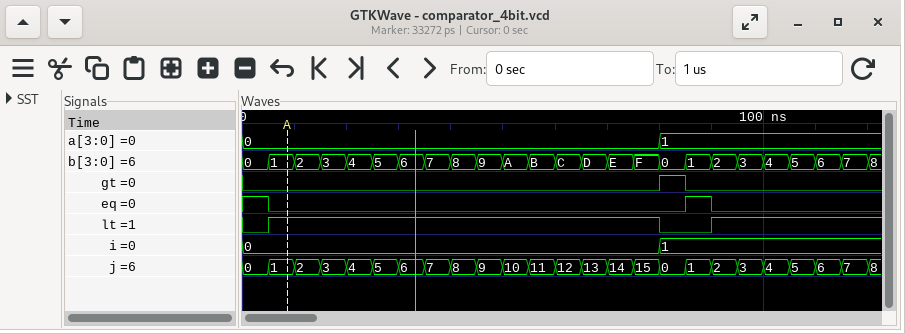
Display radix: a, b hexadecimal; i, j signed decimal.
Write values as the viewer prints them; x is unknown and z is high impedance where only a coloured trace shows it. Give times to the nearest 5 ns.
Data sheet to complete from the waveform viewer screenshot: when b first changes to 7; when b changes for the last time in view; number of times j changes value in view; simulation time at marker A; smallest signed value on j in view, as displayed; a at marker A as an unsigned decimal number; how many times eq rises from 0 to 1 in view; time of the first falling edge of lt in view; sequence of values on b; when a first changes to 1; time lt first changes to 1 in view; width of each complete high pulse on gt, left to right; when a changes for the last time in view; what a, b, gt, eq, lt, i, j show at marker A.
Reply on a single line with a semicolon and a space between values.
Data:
35 ns; 120 ns; 24; 10 ns; 0; 0; 1; 80 ns; 0, 1, 2, 3, 4, 5, 6, 7, 8, 9, A, B, C, D, E, F, 0, 1, 2, 3, 4, 5, 6, 7, 8; 80 ns; 5 ns; 5 ns; 80 ns; a=0, b=1, gt=0, eq=0, lt=1, i=0, j=1
